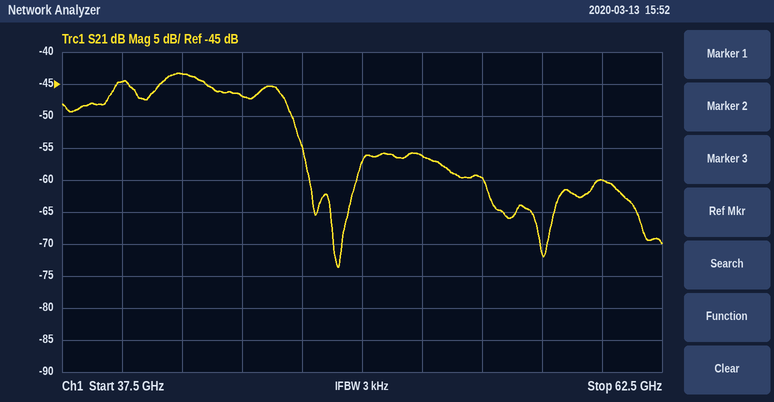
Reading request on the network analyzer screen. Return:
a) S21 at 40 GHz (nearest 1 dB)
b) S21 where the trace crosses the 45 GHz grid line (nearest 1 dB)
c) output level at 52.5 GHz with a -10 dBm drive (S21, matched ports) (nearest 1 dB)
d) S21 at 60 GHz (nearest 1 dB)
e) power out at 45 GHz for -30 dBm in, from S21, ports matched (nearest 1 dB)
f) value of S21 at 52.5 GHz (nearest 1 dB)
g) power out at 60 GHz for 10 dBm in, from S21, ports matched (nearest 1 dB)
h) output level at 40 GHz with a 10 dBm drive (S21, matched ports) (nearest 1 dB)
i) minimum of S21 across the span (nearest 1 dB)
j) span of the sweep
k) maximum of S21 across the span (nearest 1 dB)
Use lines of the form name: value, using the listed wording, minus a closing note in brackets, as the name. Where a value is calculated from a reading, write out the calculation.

S21 at 40 GHz: -45 dB
S21 where the trace crosses the 45 GHz grid line: -47 dB
output level at 52.5 GHz with a -10 dBm drive (S21, matched ports): -10 dBm + (-56 dB) = -66 dBm
S21 at 60 GHz: -60 dB
power out at 45 GHz for -30 dBm in, from S21, ports matched: -30 dBm + (-47 dB) = -77 dBm
value of S21 at 52.5 GHz: -56 dB
power out at 60 GHz for 10 dBm in, from S21, ports matched: 10 dBm + (-60 dB) = -50 dBm
output level at 40 GHz with a 10 dBm drive (S21, matched ports): 10 dBm + (-45 dB) = -35 dBm
minimum of S21 across the span: -74 dB
span of the sweep: 25 GHz
maximum of S21 across the span: -43 dB
